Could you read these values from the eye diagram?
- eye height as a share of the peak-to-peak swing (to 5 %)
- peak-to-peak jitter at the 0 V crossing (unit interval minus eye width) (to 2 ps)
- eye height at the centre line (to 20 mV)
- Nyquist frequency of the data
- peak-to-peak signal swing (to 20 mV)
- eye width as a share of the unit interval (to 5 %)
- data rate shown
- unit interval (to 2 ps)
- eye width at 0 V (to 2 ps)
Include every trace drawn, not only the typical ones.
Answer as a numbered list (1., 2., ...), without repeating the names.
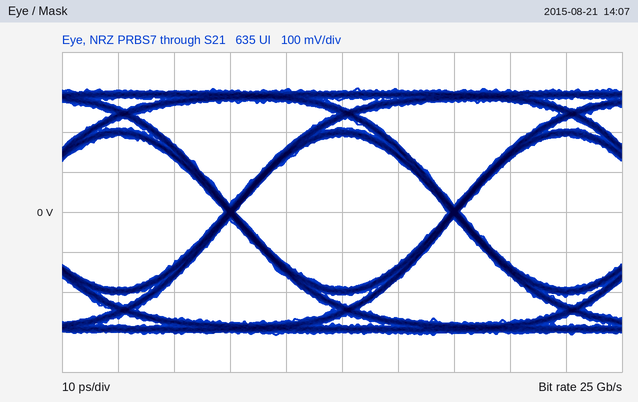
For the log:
1. 60 %
2. 2 ps
3. 380 mV
4. 12.5 GHz
5. 620 mV
6. 95 %
7. 25 Gb/s
8. 40 ps
9. 38 ps
